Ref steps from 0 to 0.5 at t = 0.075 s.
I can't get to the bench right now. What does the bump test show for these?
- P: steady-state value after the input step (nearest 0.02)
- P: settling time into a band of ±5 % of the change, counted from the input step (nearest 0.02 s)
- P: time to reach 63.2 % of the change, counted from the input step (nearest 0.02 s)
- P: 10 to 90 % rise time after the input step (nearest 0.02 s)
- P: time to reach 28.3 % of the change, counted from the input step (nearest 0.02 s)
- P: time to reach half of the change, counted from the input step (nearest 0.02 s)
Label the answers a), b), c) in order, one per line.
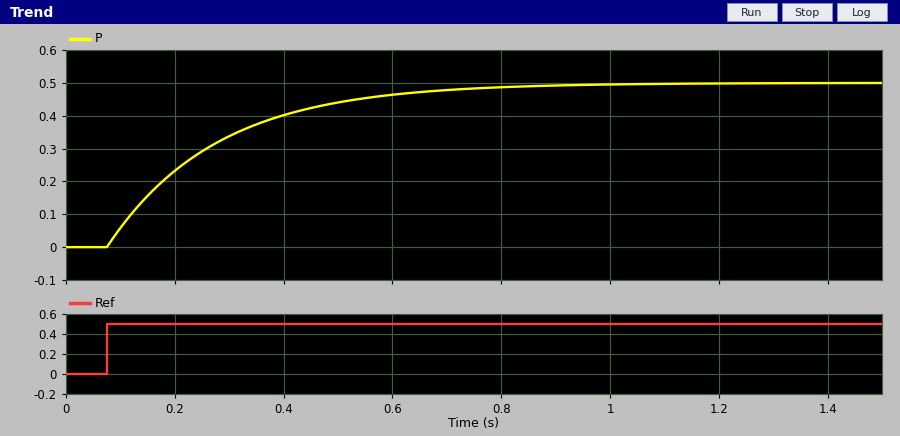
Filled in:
a) 0.50
b) 0.60 s
c) 0.20 s
d) 0.44 s
e) 0.06 s
f) 0.14 s
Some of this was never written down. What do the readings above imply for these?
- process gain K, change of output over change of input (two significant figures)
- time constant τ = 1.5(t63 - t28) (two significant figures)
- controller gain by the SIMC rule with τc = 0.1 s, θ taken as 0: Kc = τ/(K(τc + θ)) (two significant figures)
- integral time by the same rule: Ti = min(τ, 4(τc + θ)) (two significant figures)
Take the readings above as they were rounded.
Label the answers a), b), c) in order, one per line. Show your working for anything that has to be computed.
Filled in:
a) (0.5 - 0) / 0.5 = 1.0
b) 1.5 × (0.2 - 0.06) = 0.21 s
c) 0.21 / (1 × (0.1 + 0)) = 2.1
d) min(0.21, 4 × (0.1 + 0)) = 0.21 s
